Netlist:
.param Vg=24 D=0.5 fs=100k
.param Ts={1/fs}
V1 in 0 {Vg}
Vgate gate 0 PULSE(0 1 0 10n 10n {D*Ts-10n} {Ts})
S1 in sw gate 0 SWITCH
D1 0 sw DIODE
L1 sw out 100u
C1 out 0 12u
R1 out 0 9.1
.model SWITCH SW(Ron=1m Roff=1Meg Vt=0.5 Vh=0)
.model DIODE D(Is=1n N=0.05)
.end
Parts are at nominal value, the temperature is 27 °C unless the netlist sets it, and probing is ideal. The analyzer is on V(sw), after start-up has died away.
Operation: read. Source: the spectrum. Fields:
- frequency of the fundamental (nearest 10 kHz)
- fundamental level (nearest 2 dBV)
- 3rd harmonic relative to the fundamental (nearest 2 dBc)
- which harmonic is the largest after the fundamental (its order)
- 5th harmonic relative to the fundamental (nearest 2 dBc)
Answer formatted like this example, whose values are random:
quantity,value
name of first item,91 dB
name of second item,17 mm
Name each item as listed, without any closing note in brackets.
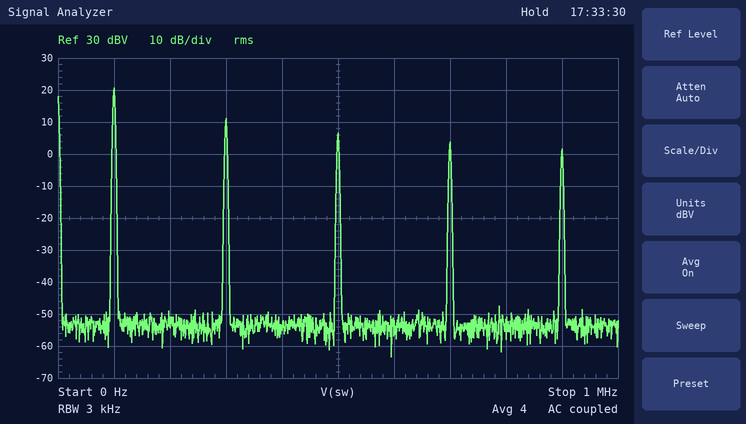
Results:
quantity,value
frequency of the fundamental,100 kHz
fundamental level,20 dBV
3rd harmonic relative to the fundamental,-10 dBc
which harmonic is the largest after the fundamental,3
5th harmonic relative to the fundamental,-14 dBc
